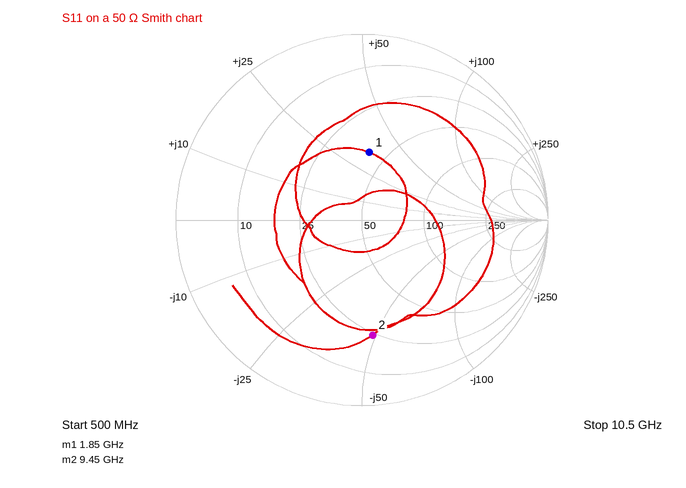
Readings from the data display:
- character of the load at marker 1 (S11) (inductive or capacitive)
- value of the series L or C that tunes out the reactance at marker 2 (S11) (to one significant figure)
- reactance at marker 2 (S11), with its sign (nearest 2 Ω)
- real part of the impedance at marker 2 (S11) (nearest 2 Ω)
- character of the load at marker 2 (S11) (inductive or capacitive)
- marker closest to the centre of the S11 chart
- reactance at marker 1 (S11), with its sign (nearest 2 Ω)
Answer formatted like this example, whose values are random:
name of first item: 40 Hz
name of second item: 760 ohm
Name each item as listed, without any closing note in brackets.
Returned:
character of the load at marker 1 (S11): inductive
value of the series L or C that tunes out the reactance at marker 2 (S11): 800 pH
reactance at marker 2 (S11), with its sign: -48 Ω
real part of the impedance at marker 2 (S11): 24 Ω
character of the load at marker 2 (S11): capacitive
marker closest to the centre of the S11 chart: marker 1
reactance at marker 1 (S11), with its sign: +34 Ω
